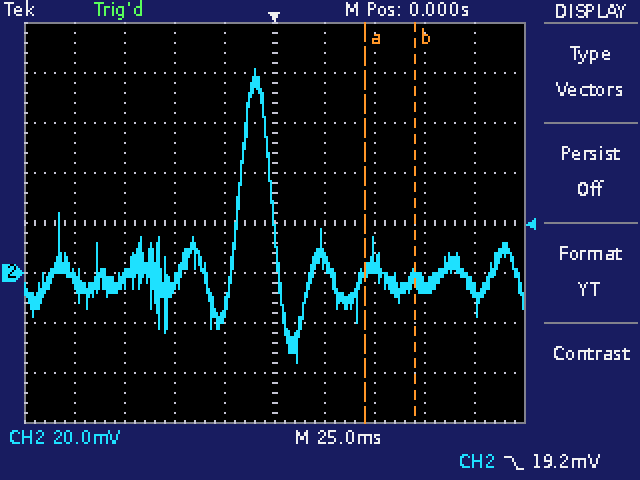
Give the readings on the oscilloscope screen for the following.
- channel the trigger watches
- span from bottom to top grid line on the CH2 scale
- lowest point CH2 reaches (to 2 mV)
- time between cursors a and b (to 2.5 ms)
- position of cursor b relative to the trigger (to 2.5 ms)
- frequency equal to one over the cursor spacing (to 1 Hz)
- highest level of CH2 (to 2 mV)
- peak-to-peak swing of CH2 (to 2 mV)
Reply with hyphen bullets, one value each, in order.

- CH2
- 160 mV
- -36 mV
- 25.0 ms
- +70.0 ms
- 40 Hz
- 82 mV
- 118 mV
